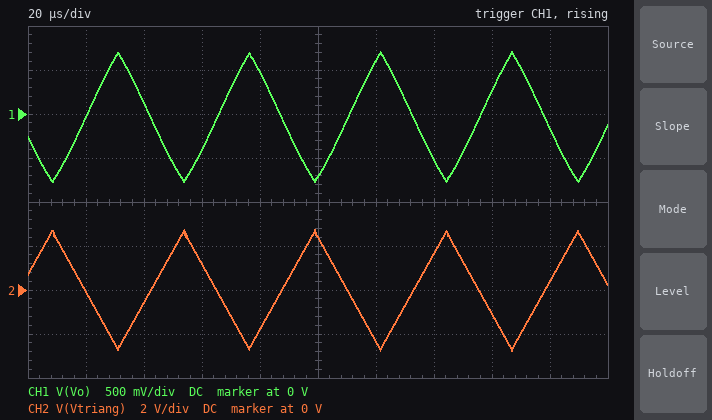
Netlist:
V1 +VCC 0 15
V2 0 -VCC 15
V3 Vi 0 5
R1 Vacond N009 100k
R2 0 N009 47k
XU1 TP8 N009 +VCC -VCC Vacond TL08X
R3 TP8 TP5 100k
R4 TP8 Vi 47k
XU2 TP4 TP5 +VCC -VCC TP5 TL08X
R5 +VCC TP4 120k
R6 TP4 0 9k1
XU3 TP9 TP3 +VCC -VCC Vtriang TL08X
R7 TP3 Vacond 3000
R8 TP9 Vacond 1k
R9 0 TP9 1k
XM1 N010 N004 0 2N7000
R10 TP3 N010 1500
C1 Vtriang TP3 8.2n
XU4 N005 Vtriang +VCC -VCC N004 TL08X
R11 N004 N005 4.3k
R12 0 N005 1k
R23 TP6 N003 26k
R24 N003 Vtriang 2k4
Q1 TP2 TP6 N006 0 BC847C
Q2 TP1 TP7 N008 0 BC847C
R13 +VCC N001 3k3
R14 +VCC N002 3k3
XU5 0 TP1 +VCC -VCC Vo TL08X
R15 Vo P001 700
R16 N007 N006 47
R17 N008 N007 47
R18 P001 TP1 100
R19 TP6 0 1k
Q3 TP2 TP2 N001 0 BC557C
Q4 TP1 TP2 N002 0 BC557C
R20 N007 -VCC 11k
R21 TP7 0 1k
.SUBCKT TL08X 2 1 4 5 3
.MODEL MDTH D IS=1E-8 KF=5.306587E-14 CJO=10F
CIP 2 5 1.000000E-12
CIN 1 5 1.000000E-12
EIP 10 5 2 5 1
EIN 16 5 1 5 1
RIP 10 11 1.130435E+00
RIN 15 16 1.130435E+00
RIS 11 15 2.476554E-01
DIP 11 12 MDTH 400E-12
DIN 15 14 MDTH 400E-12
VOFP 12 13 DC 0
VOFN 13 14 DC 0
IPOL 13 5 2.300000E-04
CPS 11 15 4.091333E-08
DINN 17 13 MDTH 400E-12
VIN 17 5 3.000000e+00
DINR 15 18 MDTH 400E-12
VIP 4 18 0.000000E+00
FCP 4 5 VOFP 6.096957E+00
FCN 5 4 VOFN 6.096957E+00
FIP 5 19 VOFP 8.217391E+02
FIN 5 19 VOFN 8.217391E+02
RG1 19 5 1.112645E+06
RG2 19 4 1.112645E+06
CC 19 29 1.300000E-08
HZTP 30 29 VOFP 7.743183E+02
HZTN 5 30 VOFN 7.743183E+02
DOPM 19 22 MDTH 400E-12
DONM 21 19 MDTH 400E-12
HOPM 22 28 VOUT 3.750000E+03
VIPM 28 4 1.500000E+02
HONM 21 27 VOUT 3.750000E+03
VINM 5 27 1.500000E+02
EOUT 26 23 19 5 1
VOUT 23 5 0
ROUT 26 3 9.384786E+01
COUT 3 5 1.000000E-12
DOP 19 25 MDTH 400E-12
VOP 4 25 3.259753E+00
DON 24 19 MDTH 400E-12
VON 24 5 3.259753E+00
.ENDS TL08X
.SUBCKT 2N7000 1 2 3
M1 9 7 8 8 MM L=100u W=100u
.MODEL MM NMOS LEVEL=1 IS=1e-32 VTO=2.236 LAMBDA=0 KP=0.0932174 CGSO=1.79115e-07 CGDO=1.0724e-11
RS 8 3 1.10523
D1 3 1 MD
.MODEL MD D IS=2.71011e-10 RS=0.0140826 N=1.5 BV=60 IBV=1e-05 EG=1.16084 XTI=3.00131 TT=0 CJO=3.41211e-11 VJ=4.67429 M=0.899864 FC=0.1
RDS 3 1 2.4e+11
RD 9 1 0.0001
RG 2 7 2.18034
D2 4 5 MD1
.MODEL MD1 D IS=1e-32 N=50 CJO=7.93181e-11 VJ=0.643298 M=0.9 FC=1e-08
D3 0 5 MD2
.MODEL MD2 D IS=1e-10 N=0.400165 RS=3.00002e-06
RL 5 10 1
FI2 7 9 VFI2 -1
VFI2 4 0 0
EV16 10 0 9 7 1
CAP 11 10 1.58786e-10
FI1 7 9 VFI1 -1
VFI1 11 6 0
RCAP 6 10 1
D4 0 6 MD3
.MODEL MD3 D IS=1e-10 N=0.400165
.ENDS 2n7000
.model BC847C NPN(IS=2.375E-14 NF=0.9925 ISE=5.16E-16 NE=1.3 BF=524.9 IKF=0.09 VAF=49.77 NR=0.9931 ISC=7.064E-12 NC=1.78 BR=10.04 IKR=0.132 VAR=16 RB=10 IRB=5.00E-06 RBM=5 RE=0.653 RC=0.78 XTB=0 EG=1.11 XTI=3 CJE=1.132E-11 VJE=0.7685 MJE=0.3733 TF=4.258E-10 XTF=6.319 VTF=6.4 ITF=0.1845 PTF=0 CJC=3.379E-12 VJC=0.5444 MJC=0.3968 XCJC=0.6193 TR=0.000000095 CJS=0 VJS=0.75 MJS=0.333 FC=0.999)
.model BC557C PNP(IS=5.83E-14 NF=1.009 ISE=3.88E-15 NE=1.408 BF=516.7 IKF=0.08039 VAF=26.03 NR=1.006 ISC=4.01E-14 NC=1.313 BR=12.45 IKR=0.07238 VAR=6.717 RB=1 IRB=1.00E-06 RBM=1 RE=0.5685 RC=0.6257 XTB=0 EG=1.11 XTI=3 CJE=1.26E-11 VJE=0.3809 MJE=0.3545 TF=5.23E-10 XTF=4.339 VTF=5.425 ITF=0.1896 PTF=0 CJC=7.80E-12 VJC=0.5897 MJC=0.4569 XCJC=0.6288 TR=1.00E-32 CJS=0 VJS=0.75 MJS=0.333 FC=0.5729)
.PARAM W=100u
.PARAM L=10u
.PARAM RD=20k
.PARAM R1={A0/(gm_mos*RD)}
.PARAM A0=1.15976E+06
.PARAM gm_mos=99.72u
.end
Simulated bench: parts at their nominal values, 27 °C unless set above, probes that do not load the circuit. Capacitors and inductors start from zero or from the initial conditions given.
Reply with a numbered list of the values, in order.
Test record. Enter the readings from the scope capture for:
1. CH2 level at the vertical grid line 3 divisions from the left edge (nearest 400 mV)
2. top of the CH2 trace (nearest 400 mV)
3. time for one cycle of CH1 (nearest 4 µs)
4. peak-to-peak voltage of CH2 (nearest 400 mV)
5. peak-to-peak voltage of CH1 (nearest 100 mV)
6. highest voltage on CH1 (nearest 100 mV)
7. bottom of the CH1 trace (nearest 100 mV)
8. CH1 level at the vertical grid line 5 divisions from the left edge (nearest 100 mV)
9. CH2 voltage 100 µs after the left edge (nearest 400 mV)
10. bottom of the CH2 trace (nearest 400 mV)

1. 1.2 V
2. 2.8 V
3. 44 µs
4. 5.6 V
5. 1.5 V
6. 700 mV
7. -800 mV
8. -700 mV
9. 2.4 V
10. -2.8 V
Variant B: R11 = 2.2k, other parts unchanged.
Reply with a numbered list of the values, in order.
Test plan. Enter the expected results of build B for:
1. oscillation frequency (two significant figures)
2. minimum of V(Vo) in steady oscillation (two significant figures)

1. 14 kHz
2. -980 mV
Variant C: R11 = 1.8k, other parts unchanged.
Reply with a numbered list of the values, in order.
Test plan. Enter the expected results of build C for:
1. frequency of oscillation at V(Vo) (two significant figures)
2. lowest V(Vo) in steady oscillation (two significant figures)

1. 13 kHz
2. -1.0 V
